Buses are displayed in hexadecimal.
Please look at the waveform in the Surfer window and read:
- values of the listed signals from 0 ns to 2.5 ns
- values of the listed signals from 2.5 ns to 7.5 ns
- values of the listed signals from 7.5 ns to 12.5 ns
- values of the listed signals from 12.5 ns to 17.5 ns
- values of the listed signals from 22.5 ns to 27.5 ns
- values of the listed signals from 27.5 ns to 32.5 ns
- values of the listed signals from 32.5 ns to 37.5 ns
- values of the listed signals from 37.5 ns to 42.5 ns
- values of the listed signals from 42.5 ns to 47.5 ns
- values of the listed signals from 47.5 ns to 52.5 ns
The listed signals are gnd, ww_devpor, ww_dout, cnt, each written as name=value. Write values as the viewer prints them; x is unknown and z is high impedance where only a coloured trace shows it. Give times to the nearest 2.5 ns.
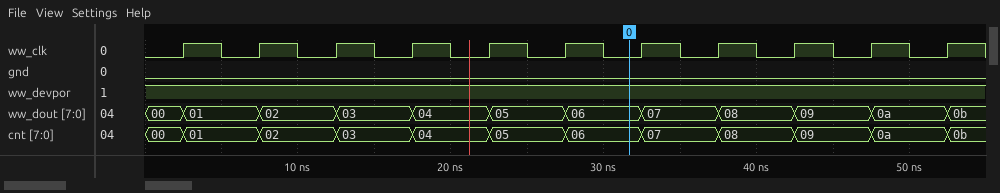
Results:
gnd=0, ww_devpor=1, ww_dout=00, cnt=00
gnd=0, ww_devpor=1, ww_dout=01, cnt=01
gnd=0, ww_devpor=1, ww_dout=02, cnt=02
gnd=0, ww_devpor=1, ww_dout=03, cnt=03
gnd=0, ww_devpor=1, ww_dout=05, cnt=05
gnd=0, ww_devpor=1, ww_dout=06, cnt=06
gnd=0, ww_devpor=1, ww_dout=07, cnt=07
gnd=0, ww_devpor=1, ww_dout=08, cnt=08
gnd=0, ww_devpor=1, ww_dout=09, cnt=09
gnd=0, ww_devpor=1, ww_dout=0a, cnt=0a
